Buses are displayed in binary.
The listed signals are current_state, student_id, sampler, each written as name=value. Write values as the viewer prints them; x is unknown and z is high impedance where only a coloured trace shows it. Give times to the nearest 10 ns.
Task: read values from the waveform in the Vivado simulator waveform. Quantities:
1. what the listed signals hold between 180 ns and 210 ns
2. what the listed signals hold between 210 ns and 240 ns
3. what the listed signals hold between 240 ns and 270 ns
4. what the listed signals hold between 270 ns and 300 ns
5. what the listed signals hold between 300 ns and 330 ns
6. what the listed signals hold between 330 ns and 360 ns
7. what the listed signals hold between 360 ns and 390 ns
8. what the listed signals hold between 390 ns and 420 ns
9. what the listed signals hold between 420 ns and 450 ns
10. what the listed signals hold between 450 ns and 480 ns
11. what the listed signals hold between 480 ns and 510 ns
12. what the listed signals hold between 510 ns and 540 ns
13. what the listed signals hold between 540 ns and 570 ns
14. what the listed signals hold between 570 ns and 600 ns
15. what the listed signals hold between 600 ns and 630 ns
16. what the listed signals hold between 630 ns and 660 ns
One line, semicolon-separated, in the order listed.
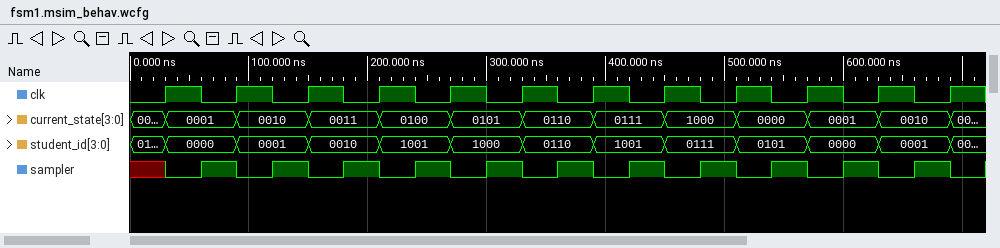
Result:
current_state=0011, student_id=0010, sampler=1; current_state=0100, student_id=1001, sampler=0; current_state=0100, student_id=1001, sampler=1; current_state=0101, student_id=1000, sampler=0; current_state=0101, student_id=1000, sampler=1; current_state=0110, student_id=0110, sampler=0; current_state=0110, student_id=0110, sampler=1; current_state=0111, student_id=1001, sampler=0; current_state=0111, student_id=1001, sampler=1; current_state=1000, student_id=0111, sampler=0; current_state=1000, student_id=0111, sampler=1; current_state=0000, student_id=0101, sampler=0; current_state=0000, student_id=0101, sampler=1; current_state=0001, student_id=0000, sampler=0; current_state=0001, student_id=0000, sampler=1; current_state=0010, student_id=0001, sampler=0
